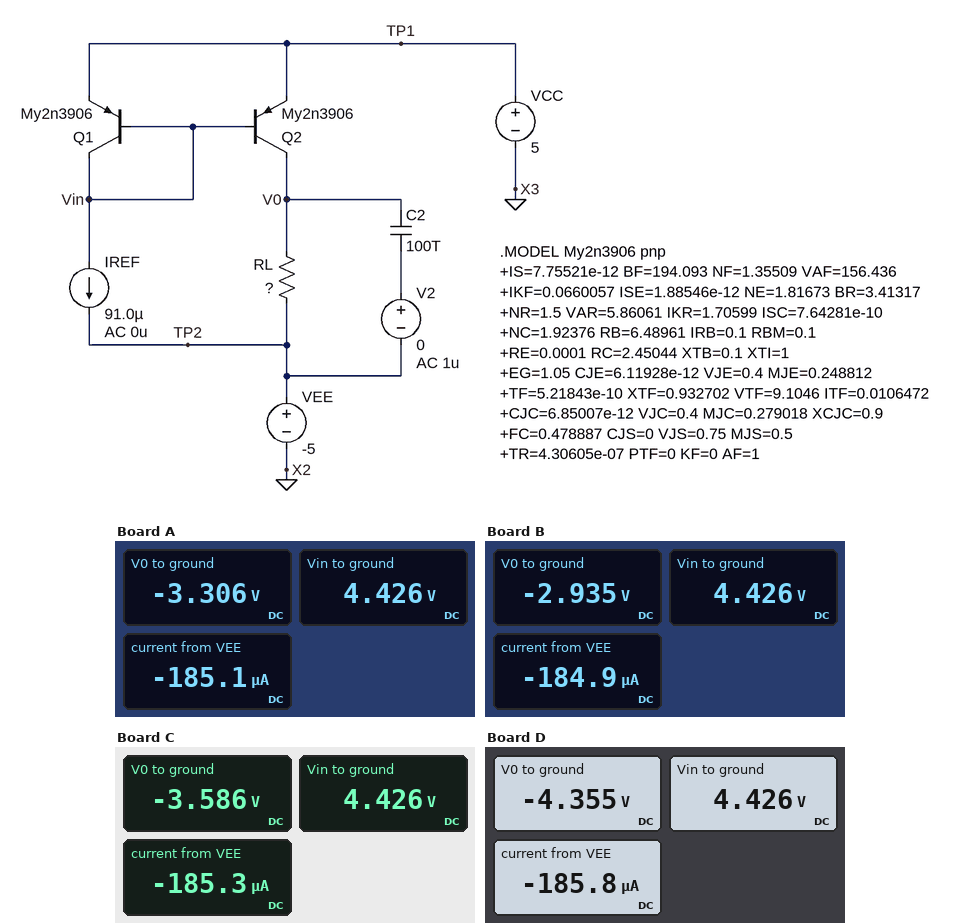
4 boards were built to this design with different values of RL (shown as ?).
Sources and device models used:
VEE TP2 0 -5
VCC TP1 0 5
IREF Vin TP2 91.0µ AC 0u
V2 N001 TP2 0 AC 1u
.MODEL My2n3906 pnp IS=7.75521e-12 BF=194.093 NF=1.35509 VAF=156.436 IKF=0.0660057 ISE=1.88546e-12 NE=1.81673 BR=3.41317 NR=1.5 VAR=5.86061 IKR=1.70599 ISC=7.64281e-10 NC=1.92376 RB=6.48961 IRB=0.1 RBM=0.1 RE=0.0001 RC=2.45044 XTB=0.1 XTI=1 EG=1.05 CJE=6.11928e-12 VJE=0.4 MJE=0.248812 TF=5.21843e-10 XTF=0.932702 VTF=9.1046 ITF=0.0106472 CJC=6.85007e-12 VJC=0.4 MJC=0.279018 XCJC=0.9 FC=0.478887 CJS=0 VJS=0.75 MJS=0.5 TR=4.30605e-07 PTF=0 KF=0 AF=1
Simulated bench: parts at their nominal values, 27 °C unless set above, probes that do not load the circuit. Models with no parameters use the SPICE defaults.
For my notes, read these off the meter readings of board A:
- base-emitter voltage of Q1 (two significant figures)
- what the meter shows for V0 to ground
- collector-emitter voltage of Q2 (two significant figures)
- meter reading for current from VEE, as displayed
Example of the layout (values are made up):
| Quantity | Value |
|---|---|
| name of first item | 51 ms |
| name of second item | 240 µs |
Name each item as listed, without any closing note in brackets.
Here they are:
| Quantity | Value |
|---|---|
| base-emitter voltage of Q1 | -570 mV |
| what the meter shows for V0 to ground | -3.306 V |
| collector-emitter voltage of Q2 | -8.3 V |
| meter reading for current from VEE, as displayed | -185.1 µA |
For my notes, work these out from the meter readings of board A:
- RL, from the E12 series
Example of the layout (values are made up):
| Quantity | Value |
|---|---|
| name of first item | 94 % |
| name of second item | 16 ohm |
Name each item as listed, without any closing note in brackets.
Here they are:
| Quantity | Value |
|---|---|
| RL, from the E12 series | 18 kΩ |
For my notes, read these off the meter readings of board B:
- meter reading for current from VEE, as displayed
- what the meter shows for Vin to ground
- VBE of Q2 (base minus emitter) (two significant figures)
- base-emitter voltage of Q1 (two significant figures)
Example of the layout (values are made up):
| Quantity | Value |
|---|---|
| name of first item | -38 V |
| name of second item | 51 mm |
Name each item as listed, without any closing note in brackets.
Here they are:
| Quantity | Value |
|---|---|
| meter reading for current from VEE, as displayed | -184.9 µA |
| what the meter shows for Vin to ground | 4.426 V |
| VBE of Q2 (base minus emitter) | -570 mV |
| base-emitter voltage of Q1 | -570 mV |
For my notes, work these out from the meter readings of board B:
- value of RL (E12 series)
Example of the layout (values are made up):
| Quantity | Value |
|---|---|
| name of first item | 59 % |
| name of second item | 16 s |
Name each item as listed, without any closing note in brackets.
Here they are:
| Quantity | Value |
|---|---|
| value of RL | 22 kΩ |
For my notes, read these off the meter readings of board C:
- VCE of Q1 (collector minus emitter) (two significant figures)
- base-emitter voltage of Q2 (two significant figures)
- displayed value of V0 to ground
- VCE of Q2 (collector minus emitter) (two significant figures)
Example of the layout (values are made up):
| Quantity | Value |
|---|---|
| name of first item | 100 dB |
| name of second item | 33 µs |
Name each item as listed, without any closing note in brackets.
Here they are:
| Quantity | Value |
|---|---|
| VCE of Q1 (collector minus emitter) | -570 mV |
| base-emitter voltage of Q2 | -570 mV |
| displayed value of V0 to ground | -3.586 V |
| VCE of Q2 (collector minus emitter) | -8.6 V |
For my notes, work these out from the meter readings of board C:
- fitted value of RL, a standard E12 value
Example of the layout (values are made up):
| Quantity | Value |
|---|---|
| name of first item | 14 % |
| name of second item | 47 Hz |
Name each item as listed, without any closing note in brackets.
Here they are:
| Quantity | Value |
|---|---|
| fitted value of RL, a standard E12 value | 15 kΩ |
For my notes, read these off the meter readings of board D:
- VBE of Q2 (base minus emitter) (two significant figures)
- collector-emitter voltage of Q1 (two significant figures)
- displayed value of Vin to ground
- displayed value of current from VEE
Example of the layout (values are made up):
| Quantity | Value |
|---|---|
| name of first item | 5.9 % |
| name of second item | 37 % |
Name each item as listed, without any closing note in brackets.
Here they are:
| Quantity | Value |
|---|---|
| VBE of Q2 (base minus emitter) | -570 mV |
| collector-emitter voltage of Q1 | -570 mV |
| displayed value of Vin to ground | 4.426 V |
| displayed value of current from VEE | -185.8 µA |
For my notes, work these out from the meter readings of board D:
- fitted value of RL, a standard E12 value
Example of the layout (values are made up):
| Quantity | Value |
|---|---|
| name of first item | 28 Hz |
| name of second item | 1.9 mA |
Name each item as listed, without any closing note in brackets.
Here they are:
| Quantity | Value |
|---|---|
| fitted value of RL, a standard E12 value | 6.8 kΩ |
